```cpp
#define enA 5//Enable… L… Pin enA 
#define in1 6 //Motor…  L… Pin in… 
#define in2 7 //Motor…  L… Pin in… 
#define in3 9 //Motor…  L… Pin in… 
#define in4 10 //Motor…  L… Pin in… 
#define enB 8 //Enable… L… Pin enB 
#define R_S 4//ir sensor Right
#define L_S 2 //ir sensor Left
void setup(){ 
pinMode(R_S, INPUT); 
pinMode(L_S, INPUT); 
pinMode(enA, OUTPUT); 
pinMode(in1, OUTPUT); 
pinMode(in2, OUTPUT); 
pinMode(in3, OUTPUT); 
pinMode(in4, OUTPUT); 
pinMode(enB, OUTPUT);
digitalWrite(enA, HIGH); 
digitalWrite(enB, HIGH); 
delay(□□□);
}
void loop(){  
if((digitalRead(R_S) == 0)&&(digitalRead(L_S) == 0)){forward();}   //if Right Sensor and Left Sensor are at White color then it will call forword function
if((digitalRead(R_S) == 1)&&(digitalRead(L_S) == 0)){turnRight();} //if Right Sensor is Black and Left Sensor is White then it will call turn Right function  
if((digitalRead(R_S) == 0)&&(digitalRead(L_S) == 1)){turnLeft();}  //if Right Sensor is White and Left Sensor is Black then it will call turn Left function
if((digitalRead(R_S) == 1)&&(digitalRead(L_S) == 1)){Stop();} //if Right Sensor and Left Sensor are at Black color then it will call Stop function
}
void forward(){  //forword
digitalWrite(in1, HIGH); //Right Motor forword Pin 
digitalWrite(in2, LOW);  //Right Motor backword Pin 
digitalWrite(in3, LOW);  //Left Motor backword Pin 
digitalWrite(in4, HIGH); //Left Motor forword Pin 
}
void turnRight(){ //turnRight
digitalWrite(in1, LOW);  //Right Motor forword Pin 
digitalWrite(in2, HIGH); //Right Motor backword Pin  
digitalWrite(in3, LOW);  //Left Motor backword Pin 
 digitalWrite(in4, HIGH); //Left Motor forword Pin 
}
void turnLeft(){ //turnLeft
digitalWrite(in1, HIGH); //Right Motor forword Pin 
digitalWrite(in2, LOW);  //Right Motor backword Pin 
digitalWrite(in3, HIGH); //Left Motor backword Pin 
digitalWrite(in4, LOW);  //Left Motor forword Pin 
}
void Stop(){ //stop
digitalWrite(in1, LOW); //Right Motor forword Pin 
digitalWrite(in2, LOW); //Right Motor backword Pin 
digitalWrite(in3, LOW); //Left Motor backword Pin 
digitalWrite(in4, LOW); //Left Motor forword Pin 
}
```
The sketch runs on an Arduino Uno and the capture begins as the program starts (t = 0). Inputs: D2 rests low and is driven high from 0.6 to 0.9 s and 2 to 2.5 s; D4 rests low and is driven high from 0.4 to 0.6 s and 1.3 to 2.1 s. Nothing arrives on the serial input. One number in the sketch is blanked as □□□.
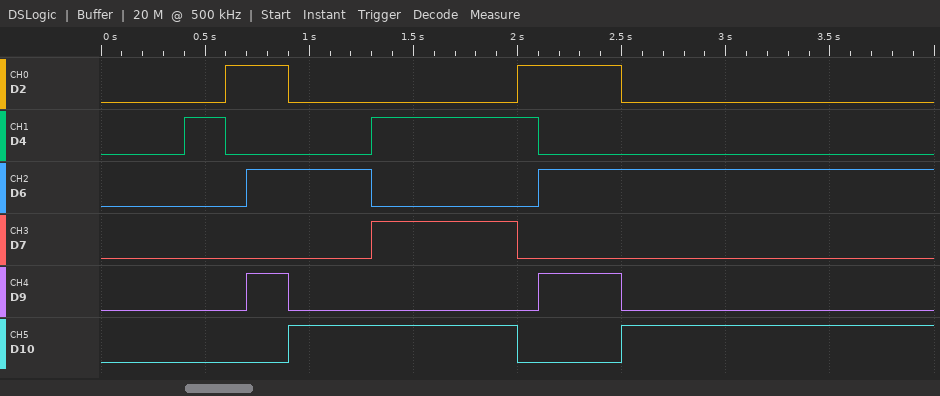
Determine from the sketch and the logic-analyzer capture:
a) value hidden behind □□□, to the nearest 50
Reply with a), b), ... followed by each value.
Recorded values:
a) 700
